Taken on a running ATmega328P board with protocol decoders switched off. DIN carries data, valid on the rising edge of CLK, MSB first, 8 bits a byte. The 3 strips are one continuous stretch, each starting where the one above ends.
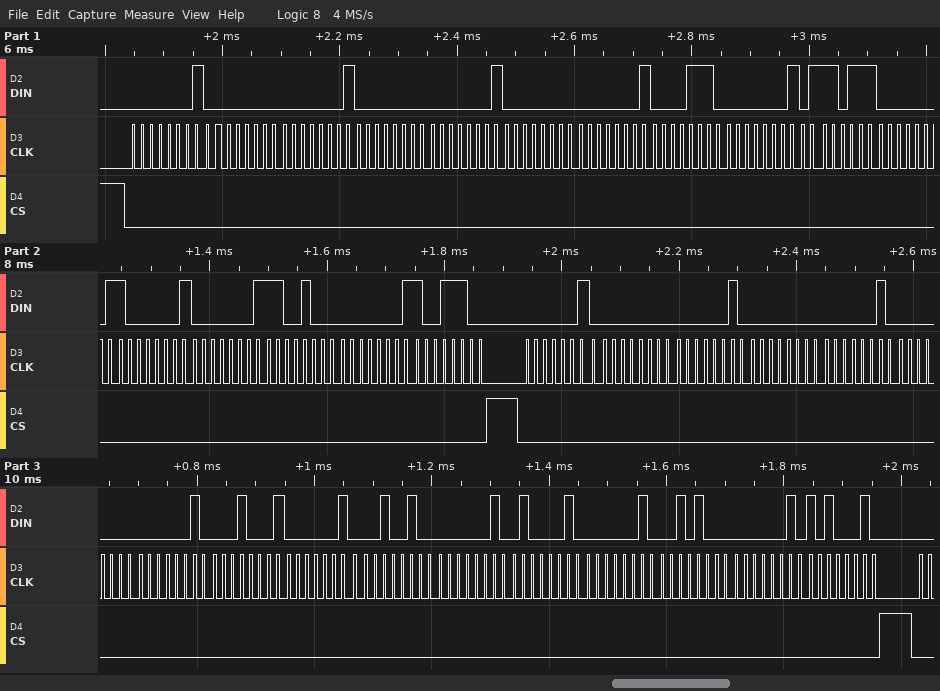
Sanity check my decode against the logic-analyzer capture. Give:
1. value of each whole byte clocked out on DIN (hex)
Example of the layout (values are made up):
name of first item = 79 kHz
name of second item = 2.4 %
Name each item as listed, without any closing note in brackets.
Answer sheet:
value of each whole byte clocked out on DIN = 01 00 01 00 01 00 01 0E 01 77 01 81 01 C8 01 9C 02 00 02 00 02 00 02 11 02 24 02 42 02 28 02 A2
